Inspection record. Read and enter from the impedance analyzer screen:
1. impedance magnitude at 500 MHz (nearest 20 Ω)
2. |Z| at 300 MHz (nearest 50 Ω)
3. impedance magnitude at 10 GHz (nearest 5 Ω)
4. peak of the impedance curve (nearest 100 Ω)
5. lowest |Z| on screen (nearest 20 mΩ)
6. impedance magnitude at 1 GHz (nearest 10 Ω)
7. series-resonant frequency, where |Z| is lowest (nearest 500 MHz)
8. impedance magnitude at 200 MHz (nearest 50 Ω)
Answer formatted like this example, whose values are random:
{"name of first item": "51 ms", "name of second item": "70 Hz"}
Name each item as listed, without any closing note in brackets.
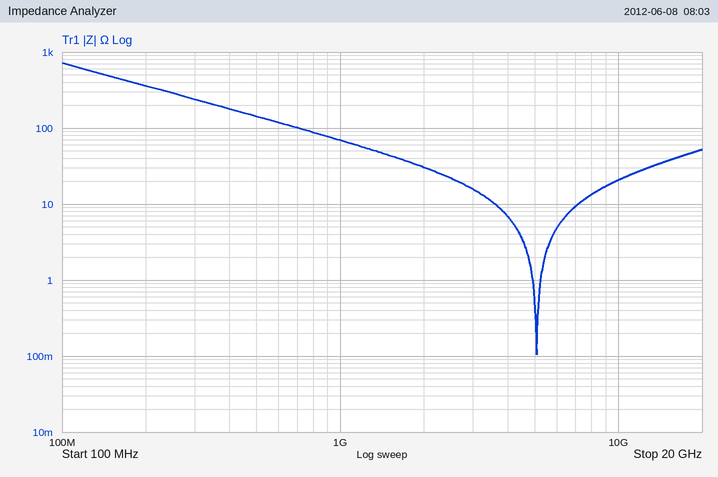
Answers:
{"impedance magnitude at 500 MHz": "140 Ω", "|Z| at 300 MHz": "250 Ω", "impedance magnitude at 10 GHz": "20 Ω", "peak of the impedance curve": "700 Ω", "lowest |Z| on screen": "100 mΩ", "impedance magnitude at 1 GHz": "70 Ω", "series-resonant frequency, where |Z| is lowest": "5.0 GHz", "impedance magnitude at 200 MHz": "350 Ω"}
